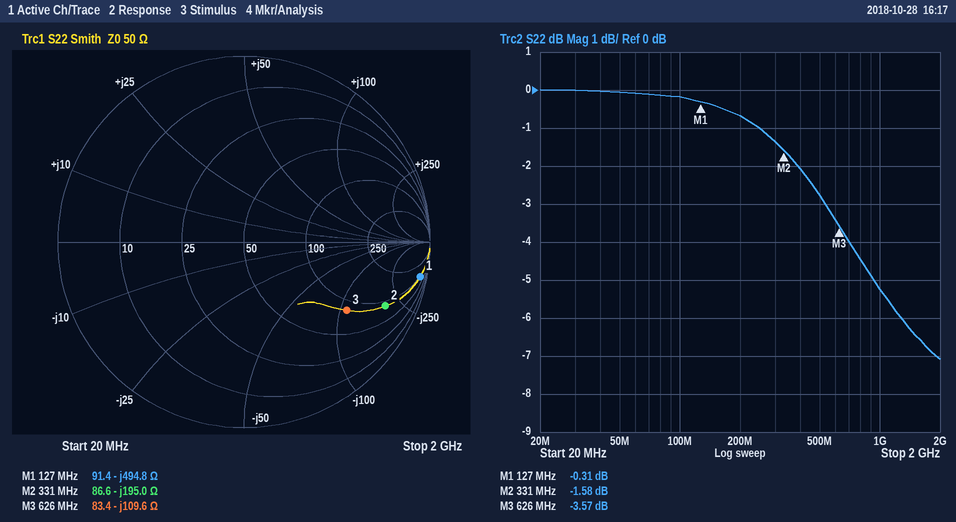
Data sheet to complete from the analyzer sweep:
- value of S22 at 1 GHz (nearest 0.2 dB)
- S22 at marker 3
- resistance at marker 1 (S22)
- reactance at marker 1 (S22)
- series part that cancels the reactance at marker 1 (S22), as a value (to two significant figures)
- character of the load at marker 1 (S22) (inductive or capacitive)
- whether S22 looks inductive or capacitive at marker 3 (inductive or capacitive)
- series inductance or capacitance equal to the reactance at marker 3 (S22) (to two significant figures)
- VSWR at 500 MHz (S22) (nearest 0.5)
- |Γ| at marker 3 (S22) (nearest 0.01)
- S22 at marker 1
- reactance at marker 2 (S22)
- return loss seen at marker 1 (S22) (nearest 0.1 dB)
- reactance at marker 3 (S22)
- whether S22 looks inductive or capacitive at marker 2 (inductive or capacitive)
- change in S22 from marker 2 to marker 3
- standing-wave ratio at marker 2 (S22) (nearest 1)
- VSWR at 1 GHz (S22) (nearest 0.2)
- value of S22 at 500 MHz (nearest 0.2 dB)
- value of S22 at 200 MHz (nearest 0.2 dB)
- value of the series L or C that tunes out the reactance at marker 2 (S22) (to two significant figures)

-5.2 dB
-3.57 dB
91.4 Ω
-494.8 Ω
620 nH
capacitive
capacitive
2.3 pF
6.5
0.66
-0.31 dB
-195.0 Ω
0.3 dB
-109.6 Ω
capacitive
-1.99 dB
11
3.4
-2.8 dB
-0.6 dB
94 nH
